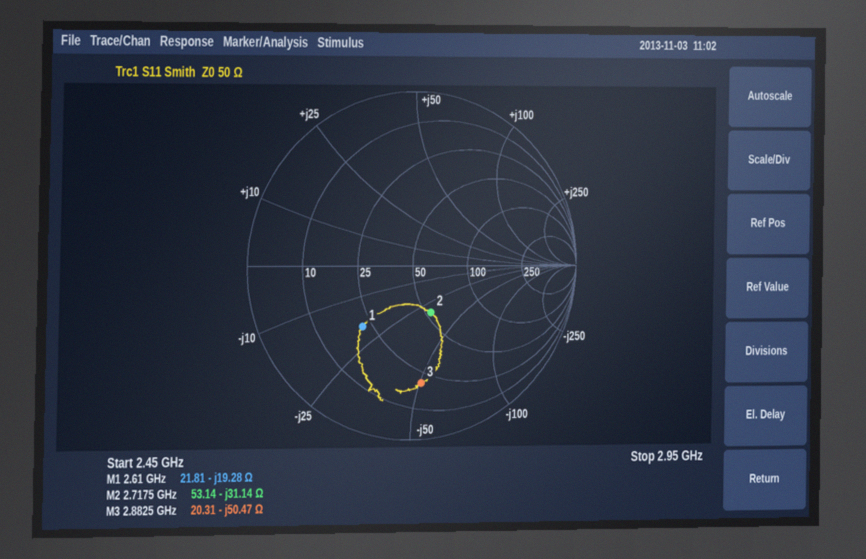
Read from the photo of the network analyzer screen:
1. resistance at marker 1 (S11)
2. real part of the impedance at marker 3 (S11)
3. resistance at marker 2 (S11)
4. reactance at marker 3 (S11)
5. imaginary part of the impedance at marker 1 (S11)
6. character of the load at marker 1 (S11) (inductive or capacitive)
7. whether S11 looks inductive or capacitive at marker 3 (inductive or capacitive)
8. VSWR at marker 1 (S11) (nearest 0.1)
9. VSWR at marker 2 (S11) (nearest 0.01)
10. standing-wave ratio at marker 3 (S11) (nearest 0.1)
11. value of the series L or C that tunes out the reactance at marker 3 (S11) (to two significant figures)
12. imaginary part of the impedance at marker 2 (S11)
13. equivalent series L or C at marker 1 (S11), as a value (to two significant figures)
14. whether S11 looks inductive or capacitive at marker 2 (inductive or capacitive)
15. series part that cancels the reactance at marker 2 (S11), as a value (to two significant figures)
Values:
21.81 Ω
20.31 Ω
53.14 Ω
-50.47 Ω
-19.28 Ω
capacitive
capacitive
2.7
1.82
5.2
2.8 nH
-31.14 Ω
3.2 pF
capacitive
1.8 nH
